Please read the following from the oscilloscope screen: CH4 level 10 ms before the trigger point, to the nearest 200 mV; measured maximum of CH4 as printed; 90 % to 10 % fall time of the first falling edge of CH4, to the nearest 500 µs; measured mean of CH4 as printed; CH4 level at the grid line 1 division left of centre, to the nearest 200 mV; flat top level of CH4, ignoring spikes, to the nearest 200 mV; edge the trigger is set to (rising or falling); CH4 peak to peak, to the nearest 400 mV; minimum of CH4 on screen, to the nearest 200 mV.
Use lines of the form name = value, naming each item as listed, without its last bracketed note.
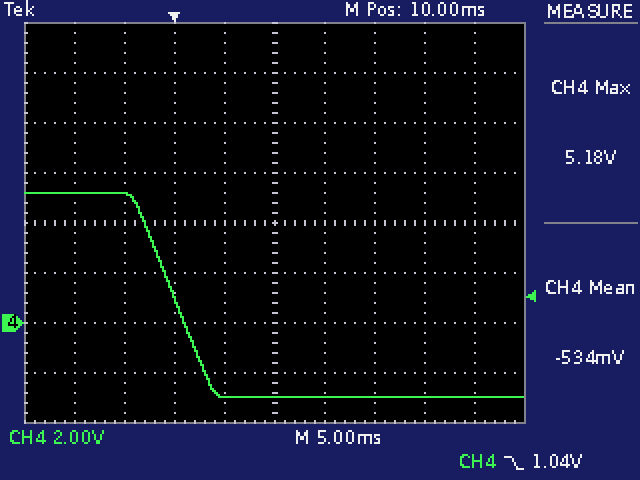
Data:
CH4 level 10 ms before the trigger point, to the nearest 200 mV = 5.2 V
measured maximum of CH4 as printed = 5.18 V
90 % to 10 % fall time of the first falling edge of CH4, to the nearest 500 µs = 6.5 ms
measured mean of CH4 as printed = -534 mV
CH4 level at the grid line 1 division left of centre, to the nearest 200 mV = -3.0 V
flat top level of CH4, ignoring spikes, to the nearest 200 mV = 5.2 V
edge the trigger is set to = falling
CH4 peak to peak, to the nearest 400 mV = 8.0 V
minimum of CH4 on screen, to the nearest 200 mV = -3.0 V
